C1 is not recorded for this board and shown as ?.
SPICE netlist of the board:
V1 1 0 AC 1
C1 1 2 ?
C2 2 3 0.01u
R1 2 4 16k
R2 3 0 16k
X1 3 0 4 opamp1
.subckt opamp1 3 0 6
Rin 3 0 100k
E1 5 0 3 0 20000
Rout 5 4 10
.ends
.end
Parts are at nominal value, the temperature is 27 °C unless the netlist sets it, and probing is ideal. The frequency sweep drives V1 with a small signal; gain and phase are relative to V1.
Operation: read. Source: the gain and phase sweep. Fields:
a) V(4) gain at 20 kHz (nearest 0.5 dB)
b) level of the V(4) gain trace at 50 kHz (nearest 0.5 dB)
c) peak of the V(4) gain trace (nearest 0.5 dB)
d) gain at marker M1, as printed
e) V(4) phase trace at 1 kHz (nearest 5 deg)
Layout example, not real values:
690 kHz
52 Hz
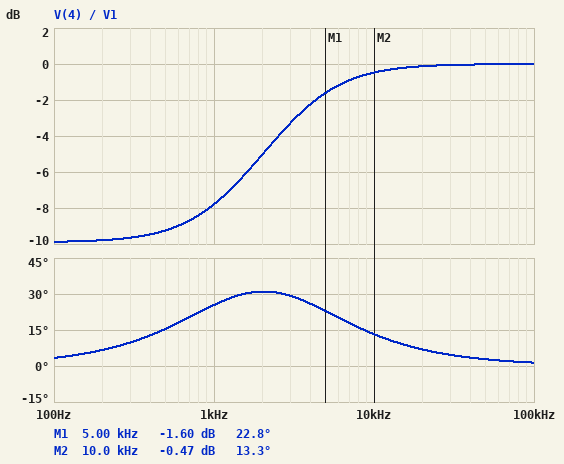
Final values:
0 dB
0 dB
0 dB
-1.60 dB
25 deg
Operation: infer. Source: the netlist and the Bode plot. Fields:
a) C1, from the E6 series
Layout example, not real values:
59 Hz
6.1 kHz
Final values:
4.7 nF
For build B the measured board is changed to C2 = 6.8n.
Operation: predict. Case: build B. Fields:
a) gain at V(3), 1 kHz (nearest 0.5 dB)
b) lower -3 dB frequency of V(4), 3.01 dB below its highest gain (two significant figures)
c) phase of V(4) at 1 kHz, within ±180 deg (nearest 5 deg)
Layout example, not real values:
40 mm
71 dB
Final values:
-12.5 dB
3.4 kHz
15 deg
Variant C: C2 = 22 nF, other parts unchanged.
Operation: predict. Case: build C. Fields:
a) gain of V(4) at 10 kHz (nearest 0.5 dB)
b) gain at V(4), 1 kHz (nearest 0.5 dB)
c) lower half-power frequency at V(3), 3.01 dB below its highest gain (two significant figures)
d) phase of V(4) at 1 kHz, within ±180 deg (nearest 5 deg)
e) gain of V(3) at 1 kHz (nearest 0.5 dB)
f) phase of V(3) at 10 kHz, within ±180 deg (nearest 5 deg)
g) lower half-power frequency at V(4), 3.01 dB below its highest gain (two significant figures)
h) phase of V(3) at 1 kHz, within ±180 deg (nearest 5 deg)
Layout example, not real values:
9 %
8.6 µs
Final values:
-0.5 dB
-9.0 dB
3.0 kHz
45 deg
-10.0 dB
15 deg
2.9 kHz
70 deg
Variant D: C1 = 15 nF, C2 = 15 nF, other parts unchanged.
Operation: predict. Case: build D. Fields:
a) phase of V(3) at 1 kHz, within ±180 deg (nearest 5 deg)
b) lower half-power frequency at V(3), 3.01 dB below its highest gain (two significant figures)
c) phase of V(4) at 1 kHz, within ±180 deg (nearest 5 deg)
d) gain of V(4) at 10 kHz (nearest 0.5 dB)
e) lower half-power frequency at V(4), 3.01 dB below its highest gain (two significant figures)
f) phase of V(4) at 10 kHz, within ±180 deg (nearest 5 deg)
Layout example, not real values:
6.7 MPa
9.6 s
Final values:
55 deg
1.5 kHz
20 deg
0 dB
1.1 kHz
5 deg
